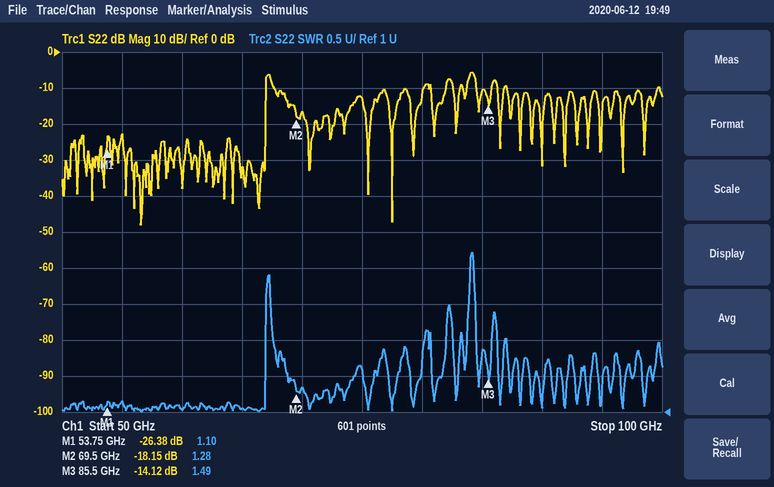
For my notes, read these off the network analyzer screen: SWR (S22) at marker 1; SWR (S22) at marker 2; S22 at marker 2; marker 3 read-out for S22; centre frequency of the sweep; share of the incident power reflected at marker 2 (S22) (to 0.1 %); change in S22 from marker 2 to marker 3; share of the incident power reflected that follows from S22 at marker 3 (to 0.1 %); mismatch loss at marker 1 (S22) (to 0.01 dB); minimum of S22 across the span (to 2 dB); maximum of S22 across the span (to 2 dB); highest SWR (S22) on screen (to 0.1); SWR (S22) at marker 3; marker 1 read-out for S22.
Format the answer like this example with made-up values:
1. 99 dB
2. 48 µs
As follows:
1. 1.10
2. 1.28
3. -18.15 dB
4. -14.12 dB
5. 75 GHz
6. 1.5 %
7. 4.03 dB
8. 3.9 %
9. 0.01 dB
10. -48 dB
11. -6 dB
12. 3.2
13. 1.49
14. -26.38 dB
